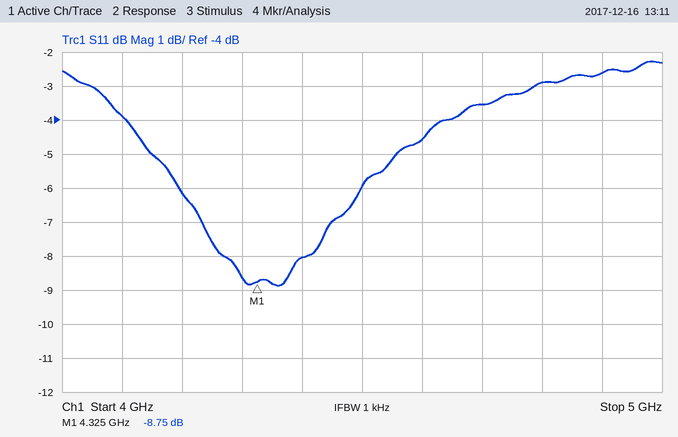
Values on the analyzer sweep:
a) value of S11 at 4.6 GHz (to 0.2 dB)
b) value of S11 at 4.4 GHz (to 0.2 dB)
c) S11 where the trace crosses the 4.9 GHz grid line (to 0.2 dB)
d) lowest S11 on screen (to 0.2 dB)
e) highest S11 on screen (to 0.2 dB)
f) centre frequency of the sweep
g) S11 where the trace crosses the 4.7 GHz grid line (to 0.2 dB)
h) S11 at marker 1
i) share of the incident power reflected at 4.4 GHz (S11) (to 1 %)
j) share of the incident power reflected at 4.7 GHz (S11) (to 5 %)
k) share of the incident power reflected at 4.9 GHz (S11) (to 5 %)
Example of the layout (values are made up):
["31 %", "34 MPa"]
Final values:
["-4.6 dB", "-8.0 dB", "-2.6 dB", "-8.8 dB", "-2.2 dB", "4.5 GHz", "-3.6 dB", "-8.75 dB", "16 %", "45 %", "55 %"]
